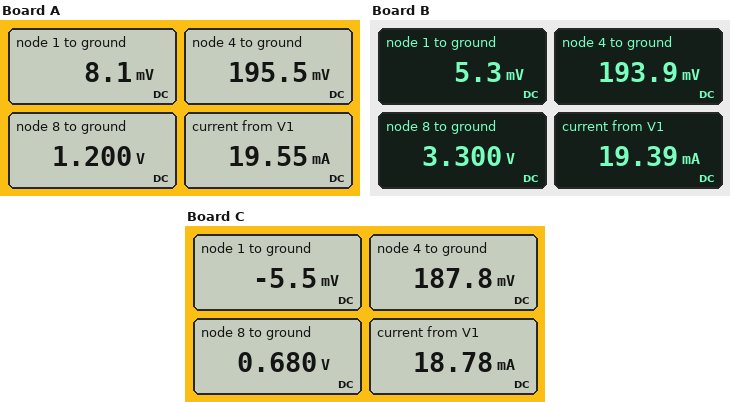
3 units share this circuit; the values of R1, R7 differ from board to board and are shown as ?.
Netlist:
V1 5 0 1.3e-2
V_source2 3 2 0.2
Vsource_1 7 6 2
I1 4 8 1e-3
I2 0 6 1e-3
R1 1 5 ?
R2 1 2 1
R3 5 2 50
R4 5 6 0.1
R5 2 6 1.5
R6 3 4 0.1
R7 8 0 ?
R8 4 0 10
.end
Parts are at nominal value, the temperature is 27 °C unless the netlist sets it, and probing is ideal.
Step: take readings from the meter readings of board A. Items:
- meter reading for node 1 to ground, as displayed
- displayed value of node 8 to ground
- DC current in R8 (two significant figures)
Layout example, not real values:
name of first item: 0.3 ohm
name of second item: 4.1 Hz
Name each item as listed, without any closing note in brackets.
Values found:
meter reading for node 1 to ground, as displayed: 8.1 mV
displayed value of node 8 to ground: 1.200 V
DC current in R8: 20 mA
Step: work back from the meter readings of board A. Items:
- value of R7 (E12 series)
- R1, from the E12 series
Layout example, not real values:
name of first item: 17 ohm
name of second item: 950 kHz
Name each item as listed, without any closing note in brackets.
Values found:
value of R7: 1.2 kΩ
R1, from the E12 series: 0.47 Ω
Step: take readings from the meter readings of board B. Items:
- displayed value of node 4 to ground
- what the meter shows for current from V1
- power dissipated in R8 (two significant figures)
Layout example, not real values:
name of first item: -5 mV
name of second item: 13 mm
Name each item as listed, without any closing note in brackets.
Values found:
displayed value of node 4 to ground: 193.9 mV
what the meter shows for current from V1: 19.39 mA
power dissipated in R8: 3.8 mW
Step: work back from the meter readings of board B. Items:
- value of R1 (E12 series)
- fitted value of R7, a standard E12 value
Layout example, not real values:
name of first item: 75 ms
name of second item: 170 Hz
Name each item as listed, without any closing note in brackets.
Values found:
value of R1: 0.82 Ω
fitted value of R7, a standard E12 value: 3.3 kΩ
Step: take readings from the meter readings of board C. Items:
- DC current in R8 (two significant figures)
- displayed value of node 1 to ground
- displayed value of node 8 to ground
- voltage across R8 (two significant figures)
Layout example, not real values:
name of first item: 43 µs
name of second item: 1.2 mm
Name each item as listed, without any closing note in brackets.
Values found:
DC current in R8: 19 mA
displayed value of node 1 to ground: -5.5 mV
displayed value of node 8 to ground: 0.680 V
voltage across R8: 190 mV
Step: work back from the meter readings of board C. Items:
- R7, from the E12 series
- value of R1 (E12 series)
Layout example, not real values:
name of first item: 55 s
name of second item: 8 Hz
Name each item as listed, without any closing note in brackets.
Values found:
R7, from the E12 series: 680 Ω
value of R1: 3.9 Ω
